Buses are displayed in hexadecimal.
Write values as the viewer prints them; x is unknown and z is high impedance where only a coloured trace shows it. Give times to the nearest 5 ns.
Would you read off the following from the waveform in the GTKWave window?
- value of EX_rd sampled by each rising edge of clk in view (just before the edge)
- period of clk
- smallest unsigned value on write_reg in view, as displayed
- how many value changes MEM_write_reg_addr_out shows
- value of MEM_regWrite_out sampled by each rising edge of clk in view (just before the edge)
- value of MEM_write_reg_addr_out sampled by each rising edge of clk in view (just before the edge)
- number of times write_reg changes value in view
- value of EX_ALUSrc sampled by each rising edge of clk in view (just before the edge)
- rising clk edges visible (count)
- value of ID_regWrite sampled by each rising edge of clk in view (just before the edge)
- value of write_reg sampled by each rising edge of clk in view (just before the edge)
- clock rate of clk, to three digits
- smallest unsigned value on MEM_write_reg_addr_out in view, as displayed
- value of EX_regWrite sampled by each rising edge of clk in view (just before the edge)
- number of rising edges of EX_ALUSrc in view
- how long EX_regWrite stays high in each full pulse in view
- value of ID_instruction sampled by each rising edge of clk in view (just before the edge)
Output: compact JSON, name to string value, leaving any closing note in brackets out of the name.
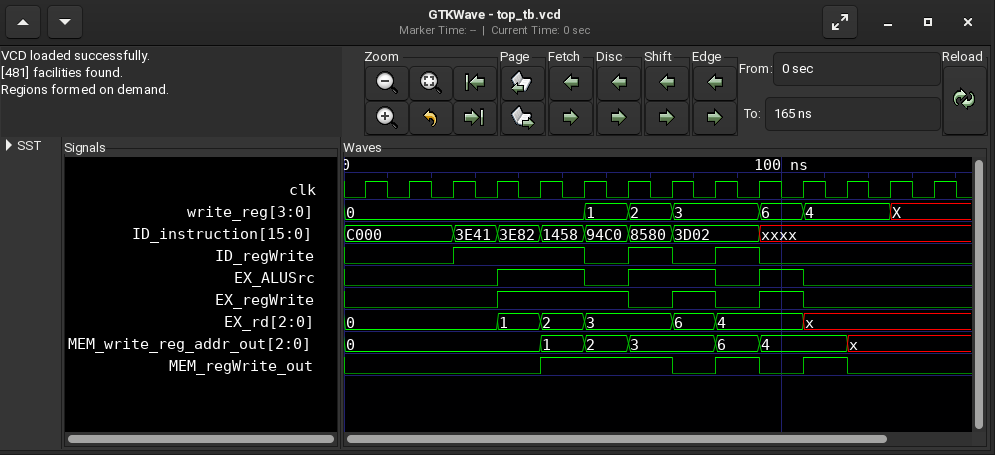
{"value of EX_rd sampled by each rising edge of clk in view": "0, 0, 0, 0, 1, 2, 3, 3, 6, 4, 4, x, x, x", "period of clk": "10 ns", "smallest unsigned value on write_reg in view, as displayed": "0", "how many value changes MEM_write_reg_addr_out shows": "6", "value of MEM_regWrite_out sampled by each rising edge of clk in view": "0 0 0 0 0 1 1 1 0 1 0 1 0 0", "value of MEM_write_reg_addr_out sampled by each rising edge of clk in view": "0, 0, 0, 0, 0, 1, 2, 3, 3, 6, 4, 4, x, x", "number of times write_reg changes value in view": "6", "value of EX_ALUSrc sampled by each rising edge of clk in view": "0 0 0 0 1 1 0 1 1 0 1 0 0 0", "rising clk edges visible": "14", "value of ID_regWrite sampled by each rising edge of clk in view": "0 0 0 1 1 1 0 1 0 1 0 0 0 0", "value of write_reg sampled by each rising edge of clk in view": "0, 0, 0, 0, 0, 0, 1, 2, 3, 3, 6, 4, 4, X", "clock rate of clk, to three digits": "100 MHz", "smallest unsigned value on MEM_write_reg_addr_out in view, as displayed": "0", "value of EX_regWrite sampled by each rising edge of clk in view": "0 0 0 0 1 1 1 0 1 0 1 0 0 0", "number of rising edges of EX_ALUSrc in view": "3", "how long EX_regWrite stays high in each full pulse in view": "30 ns, 10 ns, 10 ns", "value of ID_instruction sampled by each rising edge of clk in view": "C000, C000, C000, 3E41, 3E82, 1458, 94C0, 8580, 3D02, 3D02, xxxx, xxxx, xxxx, xxxx"}
